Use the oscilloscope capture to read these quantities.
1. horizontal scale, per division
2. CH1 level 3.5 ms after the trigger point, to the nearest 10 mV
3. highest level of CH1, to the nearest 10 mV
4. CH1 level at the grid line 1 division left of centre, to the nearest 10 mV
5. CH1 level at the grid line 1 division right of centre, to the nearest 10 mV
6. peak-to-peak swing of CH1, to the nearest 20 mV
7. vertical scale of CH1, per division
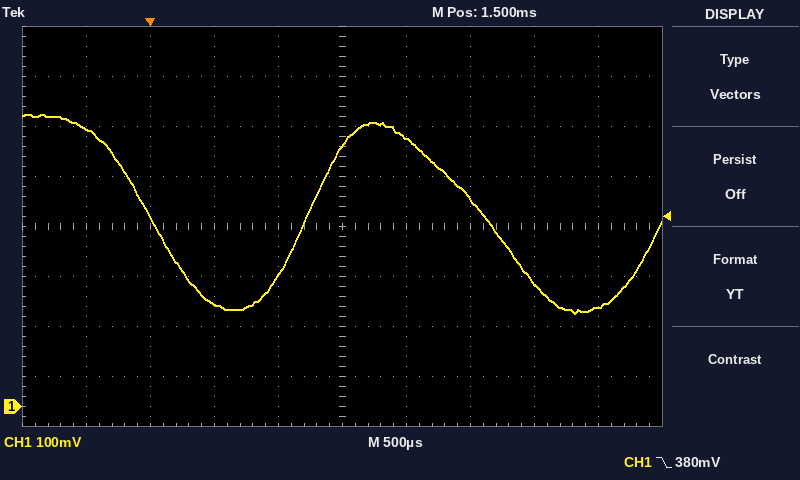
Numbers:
500 µs
200 mV
580 mV
260 mV
540 mV
400 mV
100 mV
